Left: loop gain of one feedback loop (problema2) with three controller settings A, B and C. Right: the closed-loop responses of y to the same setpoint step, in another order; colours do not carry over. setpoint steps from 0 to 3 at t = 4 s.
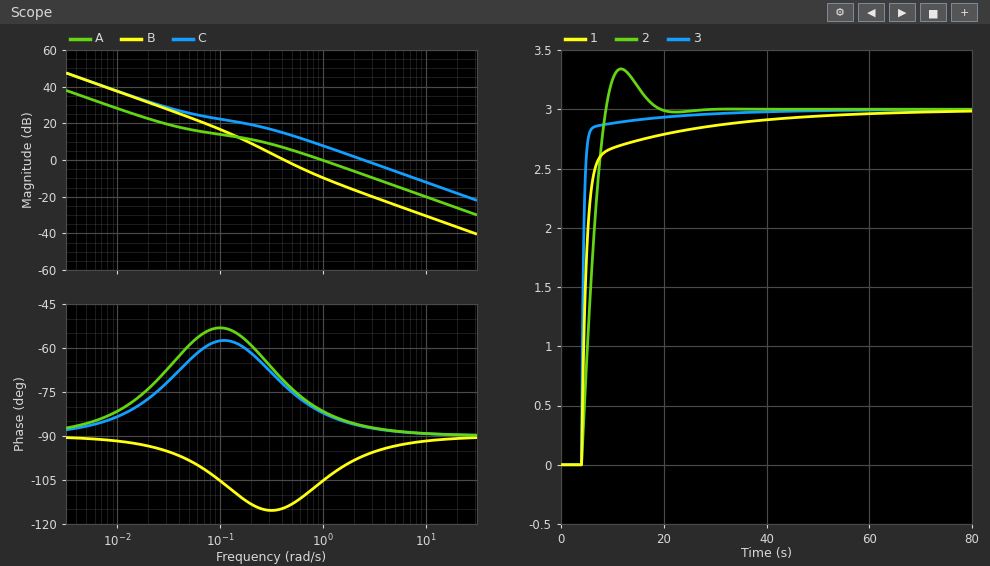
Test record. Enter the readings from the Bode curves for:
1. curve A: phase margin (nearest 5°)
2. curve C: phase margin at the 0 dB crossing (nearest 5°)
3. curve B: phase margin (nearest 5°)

100°
95°
65°
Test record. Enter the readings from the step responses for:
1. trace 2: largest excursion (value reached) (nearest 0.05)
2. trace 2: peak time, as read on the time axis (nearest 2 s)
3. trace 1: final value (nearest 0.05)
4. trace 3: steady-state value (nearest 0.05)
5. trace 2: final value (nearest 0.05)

3.35
12 s
3.00
3.00
3.00
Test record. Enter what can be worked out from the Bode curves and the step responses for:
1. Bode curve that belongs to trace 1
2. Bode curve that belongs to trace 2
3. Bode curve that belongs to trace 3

A
B
C
